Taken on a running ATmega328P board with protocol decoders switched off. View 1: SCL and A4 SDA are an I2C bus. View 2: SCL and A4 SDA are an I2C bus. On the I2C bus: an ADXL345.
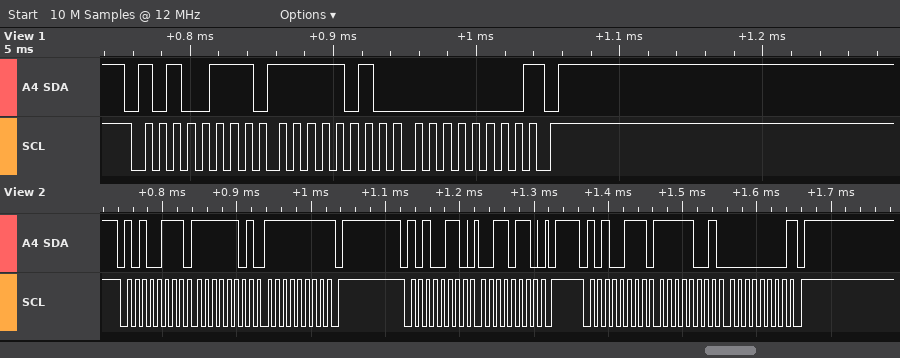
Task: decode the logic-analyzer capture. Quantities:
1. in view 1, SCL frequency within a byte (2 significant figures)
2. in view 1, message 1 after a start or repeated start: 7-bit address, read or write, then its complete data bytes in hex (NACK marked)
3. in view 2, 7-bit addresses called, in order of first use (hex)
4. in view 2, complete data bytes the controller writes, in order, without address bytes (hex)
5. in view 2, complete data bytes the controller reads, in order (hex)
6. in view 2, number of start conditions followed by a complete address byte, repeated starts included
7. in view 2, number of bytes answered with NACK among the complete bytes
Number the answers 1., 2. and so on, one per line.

1. 100 kHz
2. 0x53 read: FA 00 NACK
3. 0x53
4. 36
5. FD FF F9 00
6. 3
7. 2
